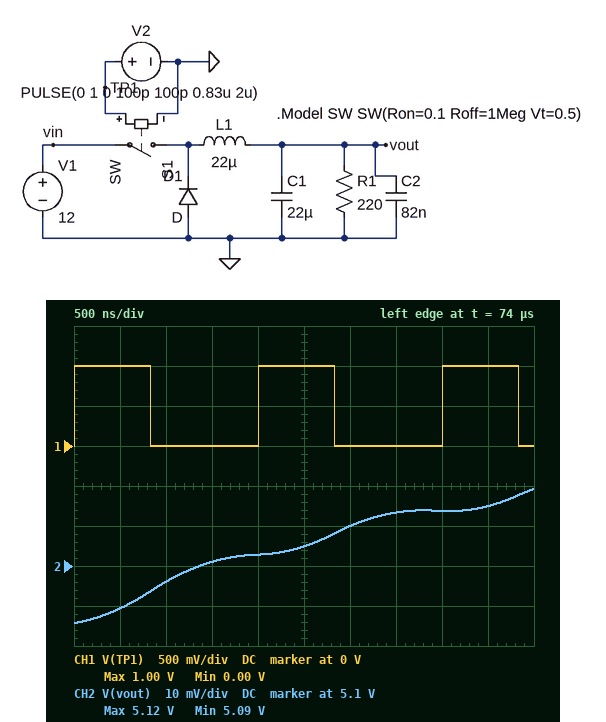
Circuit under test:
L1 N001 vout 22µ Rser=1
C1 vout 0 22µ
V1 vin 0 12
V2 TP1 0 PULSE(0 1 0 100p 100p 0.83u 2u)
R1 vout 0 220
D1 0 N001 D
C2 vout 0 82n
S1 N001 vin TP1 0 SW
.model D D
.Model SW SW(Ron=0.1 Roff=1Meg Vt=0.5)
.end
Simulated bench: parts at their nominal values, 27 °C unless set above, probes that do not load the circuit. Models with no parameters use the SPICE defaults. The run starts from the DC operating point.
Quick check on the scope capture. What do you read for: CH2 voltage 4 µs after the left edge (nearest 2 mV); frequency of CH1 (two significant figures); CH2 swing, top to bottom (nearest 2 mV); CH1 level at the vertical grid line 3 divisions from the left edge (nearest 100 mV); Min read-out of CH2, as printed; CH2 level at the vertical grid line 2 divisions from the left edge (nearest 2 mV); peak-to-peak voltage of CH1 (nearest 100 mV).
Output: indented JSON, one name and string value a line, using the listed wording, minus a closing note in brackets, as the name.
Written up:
{
  "CH2 voltage 4 µs after the left edge": "5.114 V",
  "frequency of CH1": "500 kHz",
  "CH2 swing, top to bottom": "34 mV",
  "CH1 level at the vertical grid line 3 divisions from the left edge": "0 V",
  "Min read-out of CH2, as printed": "5.09 V",
  "CH2 level at the vertical grid line 2 divisions from the left edge": "5.096 V",
  "peak-to-peak voltage of CH1": "1.0 V"
}
